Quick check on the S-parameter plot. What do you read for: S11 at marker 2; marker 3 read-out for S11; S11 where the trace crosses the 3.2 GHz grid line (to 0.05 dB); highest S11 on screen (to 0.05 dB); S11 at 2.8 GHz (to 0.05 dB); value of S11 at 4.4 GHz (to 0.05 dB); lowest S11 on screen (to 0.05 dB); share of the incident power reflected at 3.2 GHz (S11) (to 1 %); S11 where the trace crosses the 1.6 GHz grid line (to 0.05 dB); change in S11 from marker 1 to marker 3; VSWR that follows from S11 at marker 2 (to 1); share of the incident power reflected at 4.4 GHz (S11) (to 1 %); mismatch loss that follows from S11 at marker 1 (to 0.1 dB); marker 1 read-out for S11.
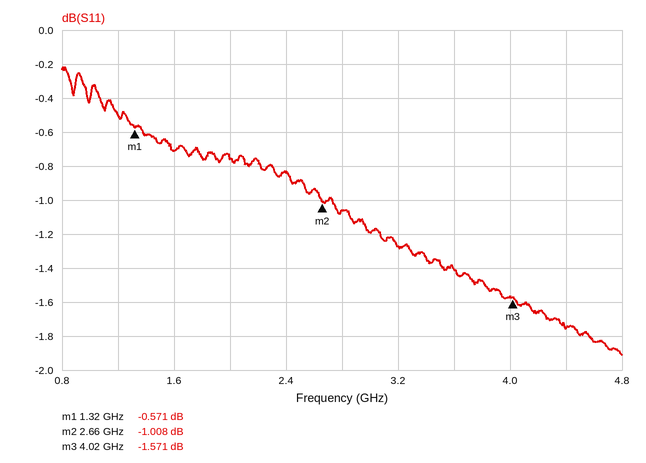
-1.008 dB
-1.571 dB
-1.25 dB
-0.20 dB
-1.05 dB
-1.75 dB
-1.90 dB
75 %
-0.70 dB
-1.000 dB
17
67 %
9.1 dB
-0.571 dB
